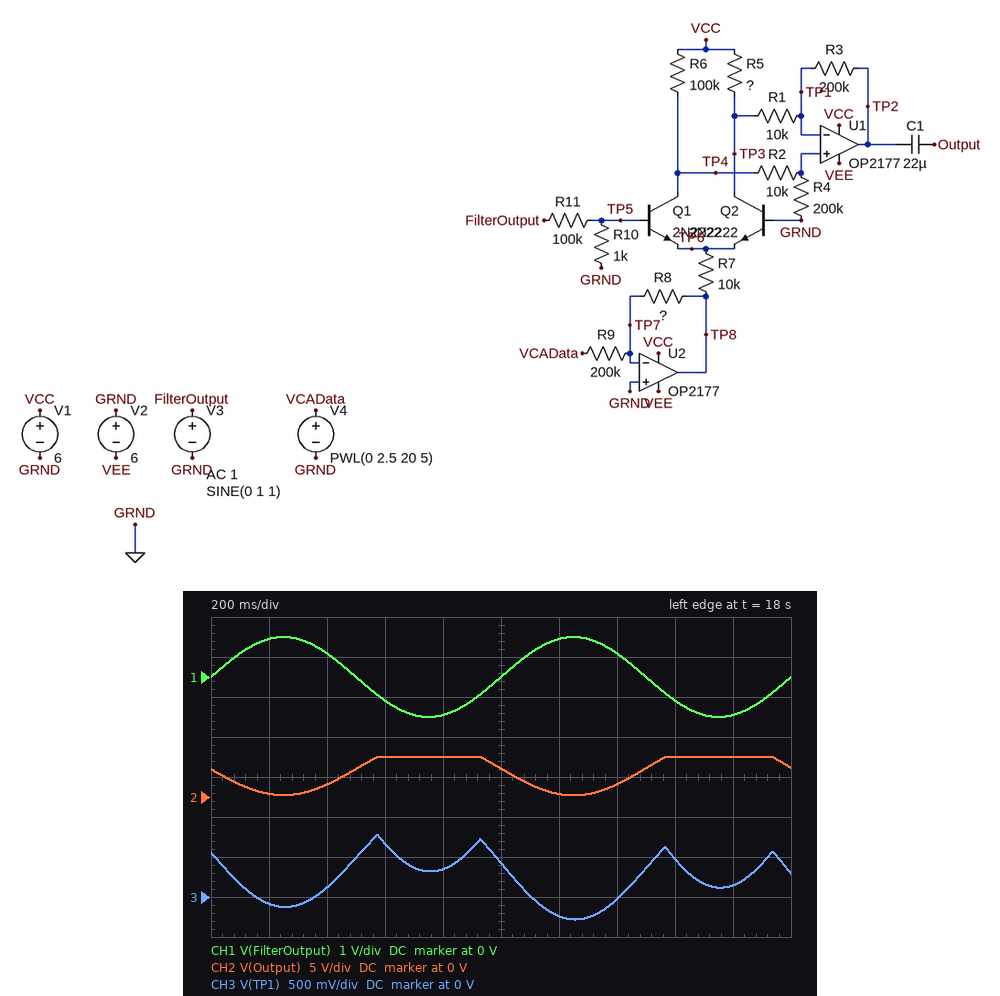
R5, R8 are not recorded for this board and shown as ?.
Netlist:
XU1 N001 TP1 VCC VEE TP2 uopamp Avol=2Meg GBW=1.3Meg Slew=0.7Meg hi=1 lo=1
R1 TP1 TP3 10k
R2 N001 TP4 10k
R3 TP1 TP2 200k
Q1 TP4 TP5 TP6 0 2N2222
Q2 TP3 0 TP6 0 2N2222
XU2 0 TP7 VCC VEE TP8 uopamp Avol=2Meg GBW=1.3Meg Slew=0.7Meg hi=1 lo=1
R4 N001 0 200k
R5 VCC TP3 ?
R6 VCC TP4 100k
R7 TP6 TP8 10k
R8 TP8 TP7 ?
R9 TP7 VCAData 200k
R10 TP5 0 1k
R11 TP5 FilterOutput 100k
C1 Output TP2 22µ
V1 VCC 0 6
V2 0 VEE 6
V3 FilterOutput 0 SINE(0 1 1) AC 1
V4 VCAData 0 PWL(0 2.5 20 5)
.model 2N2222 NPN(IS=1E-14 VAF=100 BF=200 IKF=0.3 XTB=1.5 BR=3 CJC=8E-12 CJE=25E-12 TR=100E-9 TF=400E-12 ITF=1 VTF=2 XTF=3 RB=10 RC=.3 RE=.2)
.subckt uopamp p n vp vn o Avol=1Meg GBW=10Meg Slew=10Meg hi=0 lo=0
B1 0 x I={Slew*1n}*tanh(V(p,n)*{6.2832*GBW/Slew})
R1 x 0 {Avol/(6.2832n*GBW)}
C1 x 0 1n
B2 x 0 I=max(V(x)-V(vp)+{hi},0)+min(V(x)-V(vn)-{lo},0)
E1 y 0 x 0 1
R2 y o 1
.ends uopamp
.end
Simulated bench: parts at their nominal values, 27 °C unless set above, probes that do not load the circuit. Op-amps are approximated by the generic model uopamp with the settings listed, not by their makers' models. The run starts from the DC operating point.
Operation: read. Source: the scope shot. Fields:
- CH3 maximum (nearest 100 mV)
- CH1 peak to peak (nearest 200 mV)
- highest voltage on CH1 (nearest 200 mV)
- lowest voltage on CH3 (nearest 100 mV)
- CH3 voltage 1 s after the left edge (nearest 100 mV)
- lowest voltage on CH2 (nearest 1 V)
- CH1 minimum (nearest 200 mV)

800 mV
2.0 V
1.0 V
-300 mV
400 mV
0 V
-1.0 V
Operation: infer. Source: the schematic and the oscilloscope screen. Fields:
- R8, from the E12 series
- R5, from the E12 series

68 kΩ
150 kΩ
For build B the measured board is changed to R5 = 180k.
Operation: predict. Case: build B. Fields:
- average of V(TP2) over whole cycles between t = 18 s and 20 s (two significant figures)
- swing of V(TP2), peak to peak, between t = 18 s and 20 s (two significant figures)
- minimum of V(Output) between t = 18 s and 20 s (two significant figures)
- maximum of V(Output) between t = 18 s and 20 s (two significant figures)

3.8 V
3.5 V
1.5 V
5.0 V
